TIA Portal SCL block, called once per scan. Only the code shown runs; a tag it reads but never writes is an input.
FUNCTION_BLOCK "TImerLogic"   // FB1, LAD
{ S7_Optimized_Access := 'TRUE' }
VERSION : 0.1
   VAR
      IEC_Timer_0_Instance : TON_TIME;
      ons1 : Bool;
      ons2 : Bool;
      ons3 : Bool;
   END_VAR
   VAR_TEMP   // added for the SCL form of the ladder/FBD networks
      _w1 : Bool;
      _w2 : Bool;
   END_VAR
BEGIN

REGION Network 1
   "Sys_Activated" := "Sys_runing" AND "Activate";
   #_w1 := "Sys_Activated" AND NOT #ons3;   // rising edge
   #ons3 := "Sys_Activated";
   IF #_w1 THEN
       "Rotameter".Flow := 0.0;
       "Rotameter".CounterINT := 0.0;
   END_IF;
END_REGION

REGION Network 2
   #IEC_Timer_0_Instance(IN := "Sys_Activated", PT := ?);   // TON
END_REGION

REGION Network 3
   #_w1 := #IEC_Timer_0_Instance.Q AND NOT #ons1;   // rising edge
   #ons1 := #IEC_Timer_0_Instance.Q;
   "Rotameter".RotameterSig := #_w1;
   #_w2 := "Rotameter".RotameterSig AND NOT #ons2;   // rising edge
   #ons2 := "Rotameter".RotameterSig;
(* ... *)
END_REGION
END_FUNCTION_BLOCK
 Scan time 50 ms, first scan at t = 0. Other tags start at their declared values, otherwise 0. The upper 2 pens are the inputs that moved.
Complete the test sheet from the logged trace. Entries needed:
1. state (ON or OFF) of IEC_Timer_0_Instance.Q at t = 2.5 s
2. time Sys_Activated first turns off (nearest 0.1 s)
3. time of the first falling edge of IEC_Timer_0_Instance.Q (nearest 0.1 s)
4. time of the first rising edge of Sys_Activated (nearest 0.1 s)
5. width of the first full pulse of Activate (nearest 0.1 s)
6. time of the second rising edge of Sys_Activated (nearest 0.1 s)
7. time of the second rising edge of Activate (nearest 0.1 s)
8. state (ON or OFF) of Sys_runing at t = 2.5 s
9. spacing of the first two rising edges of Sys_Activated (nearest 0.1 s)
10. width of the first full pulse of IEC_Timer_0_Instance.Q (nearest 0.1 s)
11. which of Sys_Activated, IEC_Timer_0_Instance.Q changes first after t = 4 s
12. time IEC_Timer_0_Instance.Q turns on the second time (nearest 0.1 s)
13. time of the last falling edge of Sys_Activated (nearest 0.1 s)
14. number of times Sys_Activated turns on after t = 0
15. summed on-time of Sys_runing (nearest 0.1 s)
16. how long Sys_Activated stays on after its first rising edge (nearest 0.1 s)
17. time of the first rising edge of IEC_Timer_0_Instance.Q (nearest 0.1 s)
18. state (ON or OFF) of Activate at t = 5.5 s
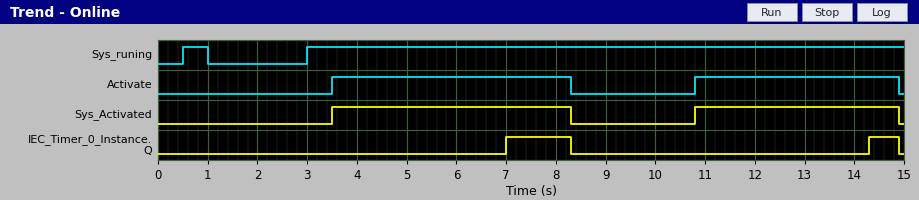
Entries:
OFF
8.3 s
8.3 s
3.5 s
4.8 s
10.8 s
10.8 s
OFF
7.3 s
1.3 s
IEC_Timer_0_Instance.Q
14.3 s
14.9 s
2
12.5 s
4.8 s
7.0 s
ON
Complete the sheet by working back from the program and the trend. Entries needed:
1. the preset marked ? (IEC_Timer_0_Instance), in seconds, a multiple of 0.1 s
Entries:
3.5 s
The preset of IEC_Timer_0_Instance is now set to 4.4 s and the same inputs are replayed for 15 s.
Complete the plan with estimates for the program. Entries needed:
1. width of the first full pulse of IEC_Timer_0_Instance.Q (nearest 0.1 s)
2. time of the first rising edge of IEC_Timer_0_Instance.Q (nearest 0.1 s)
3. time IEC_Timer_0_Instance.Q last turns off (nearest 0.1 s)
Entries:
0.4 s
7.9 s
8.3 s
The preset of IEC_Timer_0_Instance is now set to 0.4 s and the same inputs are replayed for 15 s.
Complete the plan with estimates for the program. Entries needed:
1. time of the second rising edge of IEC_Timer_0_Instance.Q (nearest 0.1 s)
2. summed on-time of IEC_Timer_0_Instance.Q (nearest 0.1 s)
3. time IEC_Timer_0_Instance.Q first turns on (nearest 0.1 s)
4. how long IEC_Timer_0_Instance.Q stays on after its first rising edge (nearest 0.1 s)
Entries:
11.2 s
8.1 s
3.9 s
4.4 s
